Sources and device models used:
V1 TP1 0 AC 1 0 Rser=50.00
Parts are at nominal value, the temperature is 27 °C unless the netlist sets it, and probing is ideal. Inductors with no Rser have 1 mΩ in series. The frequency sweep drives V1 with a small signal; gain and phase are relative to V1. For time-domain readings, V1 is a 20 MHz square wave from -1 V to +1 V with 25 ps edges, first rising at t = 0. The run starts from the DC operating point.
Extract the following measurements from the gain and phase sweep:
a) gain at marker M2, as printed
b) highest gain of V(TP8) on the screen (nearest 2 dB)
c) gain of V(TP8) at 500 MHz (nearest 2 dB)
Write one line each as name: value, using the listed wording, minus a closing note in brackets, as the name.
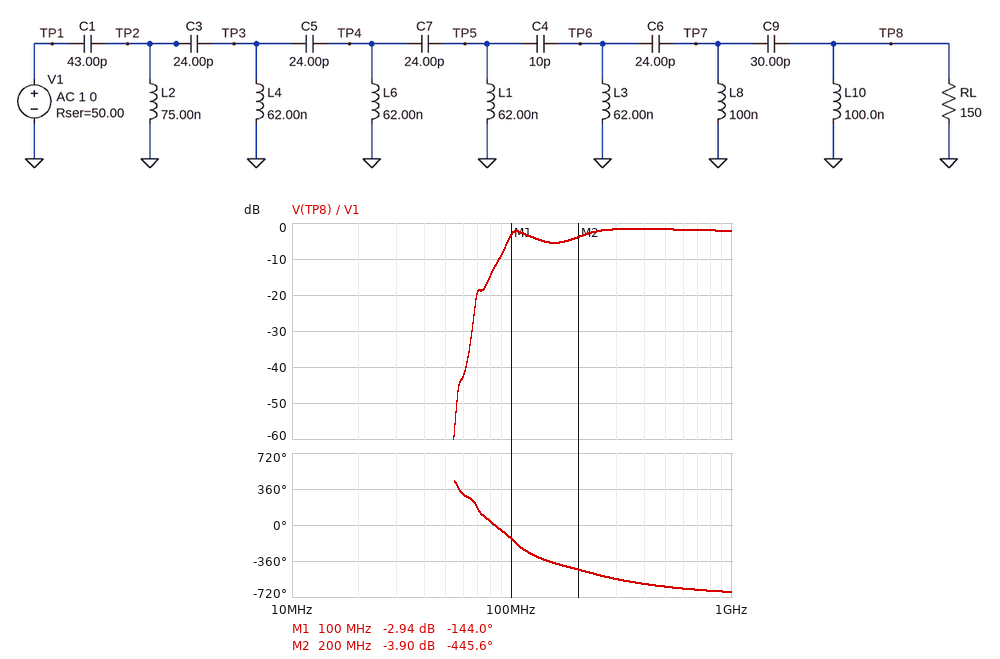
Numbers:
gain at marker M2, as printed: -3.90 dB
highest gain of V(TP8) on the screen: -2 dB
gain of V(TP8) at 500 MHz: -2 dB
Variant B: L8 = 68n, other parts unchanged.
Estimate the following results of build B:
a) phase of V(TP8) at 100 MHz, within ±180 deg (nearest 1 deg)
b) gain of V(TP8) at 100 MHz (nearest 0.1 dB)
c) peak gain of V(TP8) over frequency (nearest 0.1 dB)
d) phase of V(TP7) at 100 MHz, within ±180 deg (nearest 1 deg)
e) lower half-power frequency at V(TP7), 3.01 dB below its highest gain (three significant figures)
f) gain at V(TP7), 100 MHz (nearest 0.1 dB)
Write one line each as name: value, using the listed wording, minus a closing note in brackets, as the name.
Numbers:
phase of V(TP8) at 100 MHz, within ±180 deg: -140 deg
gain of V(TP8) at 100 MHz: -2.6 dB
peak gain of V(TP8) over frequency: -1.8 dB
phase of V(TP7) at 100 MHz, within ±180 deg: 154 deg
lower half-power frequency at V(TP7), 3.01 dB below its highest gain: 224 MHz
gain at V(TP7), 100 MHz: -10.8 dB
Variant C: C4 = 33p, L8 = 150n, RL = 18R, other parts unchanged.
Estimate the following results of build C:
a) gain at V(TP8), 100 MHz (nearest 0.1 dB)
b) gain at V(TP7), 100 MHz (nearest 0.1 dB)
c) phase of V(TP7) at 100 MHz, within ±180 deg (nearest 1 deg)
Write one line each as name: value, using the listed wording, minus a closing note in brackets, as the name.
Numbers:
gain at V(TP8), 100 MHz: -15.6 dB
gain at V(TP7), 100 MHz: -6.2 dB
phase of V(TP7) at 100 MHz, within ±180 deg: 16 deg
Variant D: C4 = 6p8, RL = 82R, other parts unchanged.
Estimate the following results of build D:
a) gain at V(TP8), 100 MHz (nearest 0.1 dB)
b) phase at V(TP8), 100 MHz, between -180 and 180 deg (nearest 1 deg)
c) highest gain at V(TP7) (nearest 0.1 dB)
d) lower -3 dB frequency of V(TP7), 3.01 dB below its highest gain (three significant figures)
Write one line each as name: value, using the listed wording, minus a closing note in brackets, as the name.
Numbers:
gain at V(TP8), 100 MHz: -11.7 dB
phase at V(TP8), 100 MHz, between -180 and 180 deg: -128 deg
highest gain at V(TP7): -4.0 dB
lower -3 dB frequency of V(TP7), 3.01 dB below its highest gain: 235 MHz
